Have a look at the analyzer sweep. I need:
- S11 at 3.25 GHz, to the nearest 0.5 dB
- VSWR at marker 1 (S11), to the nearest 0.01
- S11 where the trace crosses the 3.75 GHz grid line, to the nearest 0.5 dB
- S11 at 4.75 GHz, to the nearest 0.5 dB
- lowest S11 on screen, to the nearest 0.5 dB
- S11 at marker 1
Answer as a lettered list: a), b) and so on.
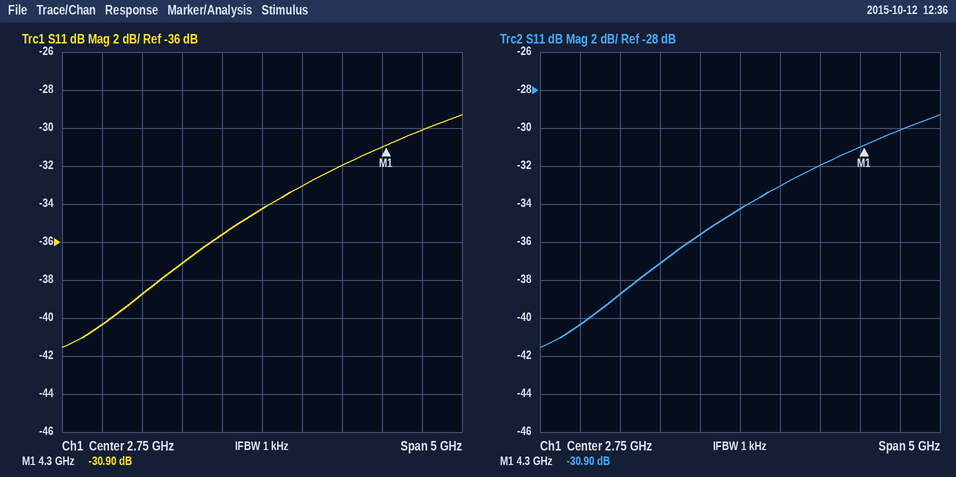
a) -33.0 dB
b) 1.06
c) -32.0 dB
d) -30.0 dB
e) -41.5 dB
f) -30.90 dB
